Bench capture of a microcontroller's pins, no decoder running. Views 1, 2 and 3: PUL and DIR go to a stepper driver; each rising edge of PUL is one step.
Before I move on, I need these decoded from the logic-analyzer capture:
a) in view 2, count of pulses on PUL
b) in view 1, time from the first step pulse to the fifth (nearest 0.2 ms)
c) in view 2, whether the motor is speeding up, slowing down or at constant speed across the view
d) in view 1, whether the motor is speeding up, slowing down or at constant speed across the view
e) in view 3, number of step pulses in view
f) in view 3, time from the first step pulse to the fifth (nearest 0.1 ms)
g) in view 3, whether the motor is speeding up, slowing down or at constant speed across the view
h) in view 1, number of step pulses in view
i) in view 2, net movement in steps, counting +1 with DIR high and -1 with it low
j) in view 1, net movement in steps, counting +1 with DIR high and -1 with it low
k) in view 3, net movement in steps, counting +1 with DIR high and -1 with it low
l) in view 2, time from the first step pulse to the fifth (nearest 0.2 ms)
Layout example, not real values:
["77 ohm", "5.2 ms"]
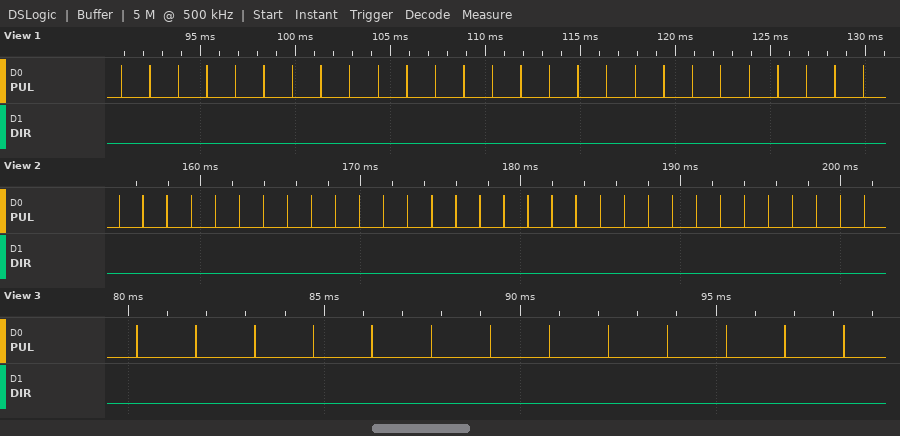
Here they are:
["32", "6.0 ms", "constant speed", "constant speed", "13", "6.0 ms", "constant speed", "27", "-32", "-27", "-13", "6.0 ms"]
